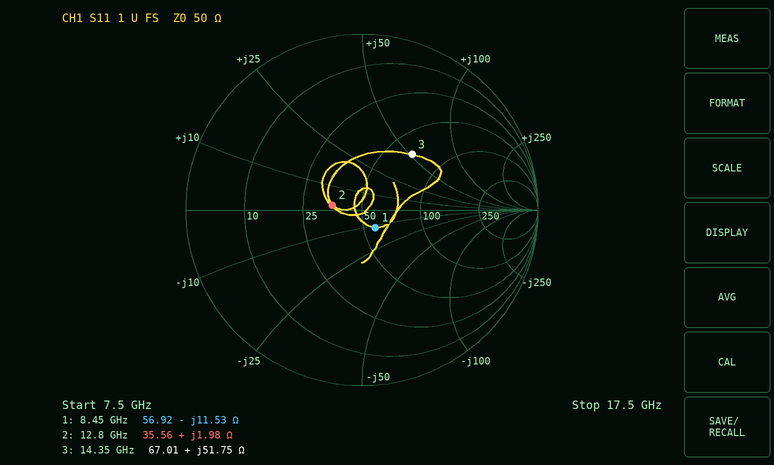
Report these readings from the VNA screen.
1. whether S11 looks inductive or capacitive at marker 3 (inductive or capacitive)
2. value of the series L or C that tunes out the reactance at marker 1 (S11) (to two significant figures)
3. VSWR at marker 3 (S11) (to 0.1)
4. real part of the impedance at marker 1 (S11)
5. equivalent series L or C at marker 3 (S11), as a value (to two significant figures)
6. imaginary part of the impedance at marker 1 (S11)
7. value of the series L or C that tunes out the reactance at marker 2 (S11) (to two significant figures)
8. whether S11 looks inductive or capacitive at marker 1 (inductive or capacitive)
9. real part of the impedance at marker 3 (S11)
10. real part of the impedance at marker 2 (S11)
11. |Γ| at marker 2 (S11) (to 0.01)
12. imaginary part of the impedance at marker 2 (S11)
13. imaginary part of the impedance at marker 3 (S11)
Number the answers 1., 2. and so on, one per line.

1. inductive
2. 220 pH
3. 2.5
4. 56.92 Ω
5. 570 pH
6. -11.53 Ω
7. 6.3 pF
8. capacitive
9. 67.01 Ω
10. 35.56 Ω
11. 0.17
12. +1.98 Ω
13. +51.75 Ω
